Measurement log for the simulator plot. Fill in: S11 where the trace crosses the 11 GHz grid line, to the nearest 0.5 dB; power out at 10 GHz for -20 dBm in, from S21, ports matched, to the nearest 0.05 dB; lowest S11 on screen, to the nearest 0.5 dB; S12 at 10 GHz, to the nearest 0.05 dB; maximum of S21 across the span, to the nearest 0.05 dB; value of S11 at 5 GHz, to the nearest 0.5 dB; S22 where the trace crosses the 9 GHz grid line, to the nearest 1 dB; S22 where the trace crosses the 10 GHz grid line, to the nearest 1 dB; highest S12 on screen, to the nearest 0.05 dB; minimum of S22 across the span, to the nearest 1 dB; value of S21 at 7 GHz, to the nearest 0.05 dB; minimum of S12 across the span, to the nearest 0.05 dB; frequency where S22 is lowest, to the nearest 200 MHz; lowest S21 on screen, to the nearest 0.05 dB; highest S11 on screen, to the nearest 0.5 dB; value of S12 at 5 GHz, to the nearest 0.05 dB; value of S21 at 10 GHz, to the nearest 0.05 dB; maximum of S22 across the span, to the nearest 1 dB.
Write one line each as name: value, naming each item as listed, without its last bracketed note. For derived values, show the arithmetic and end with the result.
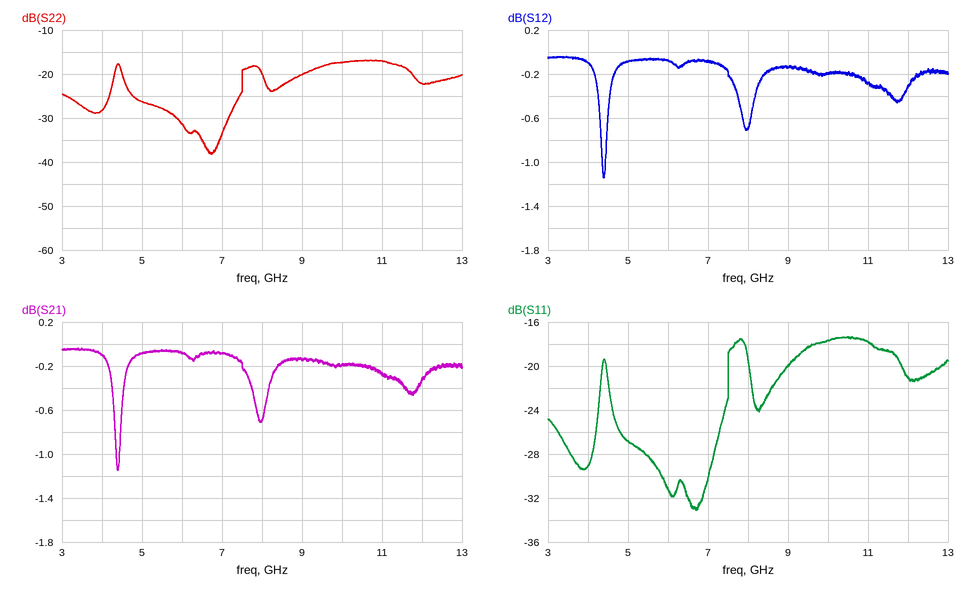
S11 where the trace crosses the 11 GHz grid line, to the nearest 0.5 dB: -18.0 dB
power out at 10 GHz for -20 dBm in, from S21, ports matched, to the nearest 0.05 dB: -20 dBm + (-0.20 dB) = -20.20 dBm
lowest S11 on screen, to the nearest 0.5 dB: -33.0 dB
S12 at 10 GHz, to the nearest 0.05 dB: -0.20 dB
maximum of S21 across the span, to the nearest 0.05 dB: -0.05 dB
value of S11 at 5 GHz, to the nearest 0.5 dB: -27.0 dB
S22 where the trace crosses the 9 GHz grid line, to the nearest 1 dB: -20 dB
S22 where the trace crosses the 10 GHz grid line, to the nearest 1 dB: -17 dB
highest S12 on screen, to the nearest 0.05 dB: -0.05 dB
minimum of S22 across the span, to the nearest 1 dB: -38 dB
value of S21 at 7 GHz, to the nearest 0.05 dB: -0.10 dB
minimum of S12 across the span, to the nearest 0.05 dB: -1.15 dB
frequency where S22 is lowest, to the nearest 200 MHz: 6.8 GHz
lowest S21 on screen, to the nearest 0.05 dB: -1.15 dB
highest S11 on screen, to the nearest 0.5 dB: -17.5 dB
value of S12 at 5 GHz, to the nearest 0.05 dB: -0.10 dB
value of S21 at 10 GHz, to the nearest 0.05 dB: -0.20 dB
maximum of S22 across the span, to the nearest 1 dB: -17 dB
